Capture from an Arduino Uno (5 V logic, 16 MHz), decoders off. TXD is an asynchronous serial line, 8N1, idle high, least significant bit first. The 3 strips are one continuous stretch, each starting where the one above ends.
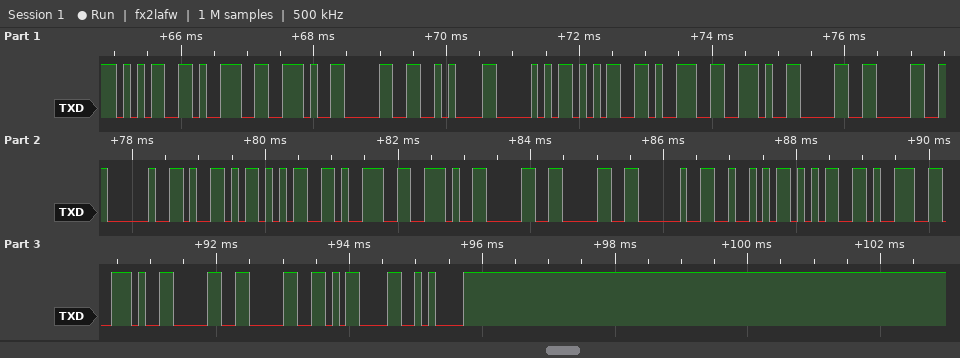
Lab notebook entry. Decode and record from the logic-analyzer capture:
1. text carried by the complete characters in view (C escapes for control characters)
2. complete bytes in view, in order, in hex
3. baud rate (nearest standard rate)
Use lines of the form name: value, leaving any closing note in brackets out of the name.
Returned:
text carried by the complete characters in view: "59.0\nP59.00 Y59.00 R59.00\r\n"
complete bytes in view, in order, in hex: 35 39 2E 30 0A 50 35 39 2E 30 30 20 59 35 39 2E 30 30 20 52 35 39 2E 30 30 0D 0A
baud rate: 9600 baud
